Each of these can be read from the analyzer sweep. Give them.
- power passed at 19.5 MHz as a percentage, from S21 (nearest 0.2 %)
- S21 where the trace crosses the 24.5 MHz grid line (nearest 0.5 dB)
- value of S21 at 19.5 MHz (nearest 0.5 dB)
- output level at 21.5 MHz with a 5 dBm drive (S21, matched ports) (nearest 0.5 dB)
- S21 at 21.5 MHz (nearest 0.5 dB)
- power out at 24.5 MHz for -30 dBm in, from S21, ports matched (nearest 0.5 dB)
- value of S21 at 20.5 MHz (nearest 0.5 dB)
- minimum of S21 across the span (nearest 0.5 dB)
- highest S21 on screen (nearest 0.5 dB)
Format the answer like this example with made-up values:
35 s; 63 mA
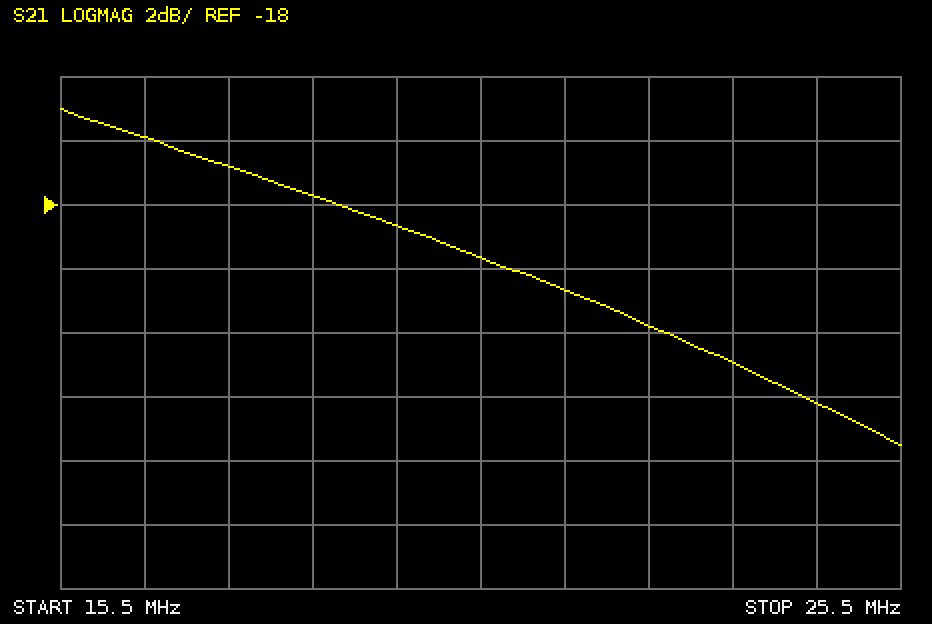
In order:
1.4 %; -24.0 dB; -18.5 dB; -15.5 dBm; -20.5 dB; -54.0 dBm; -19.5 dB; -25.5 dB; -15.0 dB
